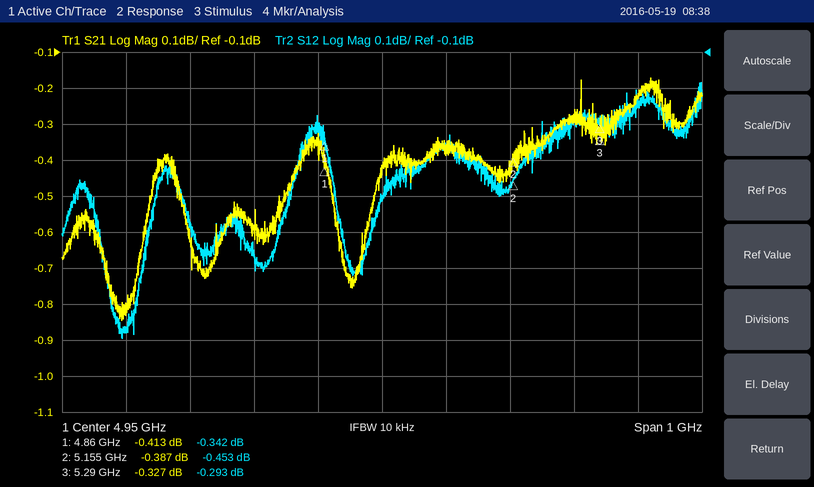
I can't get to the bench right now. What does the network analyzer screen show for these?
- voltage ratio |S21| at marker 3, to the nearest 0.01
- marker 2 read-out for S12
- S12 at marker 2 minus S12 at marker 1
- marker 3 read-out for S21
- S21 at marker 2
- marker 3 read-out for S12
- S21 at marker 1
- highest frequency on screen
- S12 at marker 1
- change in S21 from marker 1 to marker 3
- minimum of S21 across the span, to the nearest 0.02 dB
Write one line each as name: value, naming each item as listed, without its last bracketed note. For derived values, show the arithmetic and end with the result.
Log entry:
voltage ratio |S21| at marker 3, to the nearest 0.01: 10^(-0.327/20) ≈ 0.96
marker 2 read-out for S12: -0.453 dB
S12 at marker 2 minus S12 at marker 1: -0.453 − (-0.342) = -0.111 dB
marker 3 read-out for S21: -0.327 dB
S21 at marker 2: -0.387 dB
marker 3 read-out for S12: -0.293 dB
S21 at marker 1: -0.413 dB
highest frequency on screen: 5.45 GHz
S12 at marker 1: -0.342 dB
change in S21 from marker 1 to marker 3: -0.327 − (-0.413) = 0.086 dB
minimum of S21 across the span, to the nearest 0.02 dB: -0.84 dB
